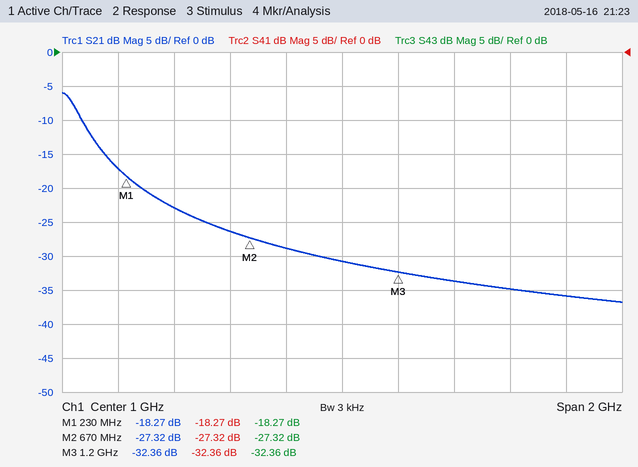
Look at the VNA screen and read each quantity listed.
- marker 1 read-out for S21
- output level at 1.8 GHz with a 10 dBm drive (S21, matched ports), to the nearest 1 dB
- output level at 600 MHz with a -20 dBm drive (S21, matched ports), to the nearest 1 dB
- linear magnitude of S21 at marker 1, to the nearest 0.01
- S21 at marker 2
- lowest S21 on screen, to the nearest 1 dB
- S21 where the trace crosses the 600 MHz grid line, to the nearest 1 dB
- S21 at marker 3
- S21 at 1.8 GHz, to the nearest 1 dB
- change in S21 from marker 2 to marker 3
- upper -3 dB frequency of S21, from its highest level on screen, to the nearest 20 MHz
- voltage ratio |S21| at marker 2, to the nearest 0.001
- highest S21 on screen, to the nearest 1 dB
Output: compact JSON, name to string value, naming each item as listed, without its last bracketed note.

{"marker 1 read-out for S21": "-18.27 dB", "output level at 1.8 GHz with a 10 dBm drive (S21, matched ports), to the nearest 1 dB": "-26 dBm", "output level at 600 MHz with a -20 dBm drive (S21, matched ports), to the nearest 1 dB": "-46 dBm", "linear magnitude of S21 at marker 1, to the nearest 0.01": "0.12", "S21 at marker 2": "-27.32 dB", "lowest S21 on screen, to the nearest 1 dB": "-37 dB", "S21 where the trace crosses the 600 MHz grid line, to the nearest 1 dB": "-26 dB", "S21 at marker 3": "-32.36 dB", "S21 at 1.8 GHz, to the nearest 1 dB": "-36 dB", "change in S21 from marker 2 to marker 3": "-5.04 dB", "upper -3 dB frequency of S21, from its highest level on screen, to the nearest 20 MHz": "60 MHz", "voltage ratio |S21| at marker 2, to the nearest 0.001": "0.043", "highest S21 on screen, to the nearest 1 dB": "-6 dB"}
